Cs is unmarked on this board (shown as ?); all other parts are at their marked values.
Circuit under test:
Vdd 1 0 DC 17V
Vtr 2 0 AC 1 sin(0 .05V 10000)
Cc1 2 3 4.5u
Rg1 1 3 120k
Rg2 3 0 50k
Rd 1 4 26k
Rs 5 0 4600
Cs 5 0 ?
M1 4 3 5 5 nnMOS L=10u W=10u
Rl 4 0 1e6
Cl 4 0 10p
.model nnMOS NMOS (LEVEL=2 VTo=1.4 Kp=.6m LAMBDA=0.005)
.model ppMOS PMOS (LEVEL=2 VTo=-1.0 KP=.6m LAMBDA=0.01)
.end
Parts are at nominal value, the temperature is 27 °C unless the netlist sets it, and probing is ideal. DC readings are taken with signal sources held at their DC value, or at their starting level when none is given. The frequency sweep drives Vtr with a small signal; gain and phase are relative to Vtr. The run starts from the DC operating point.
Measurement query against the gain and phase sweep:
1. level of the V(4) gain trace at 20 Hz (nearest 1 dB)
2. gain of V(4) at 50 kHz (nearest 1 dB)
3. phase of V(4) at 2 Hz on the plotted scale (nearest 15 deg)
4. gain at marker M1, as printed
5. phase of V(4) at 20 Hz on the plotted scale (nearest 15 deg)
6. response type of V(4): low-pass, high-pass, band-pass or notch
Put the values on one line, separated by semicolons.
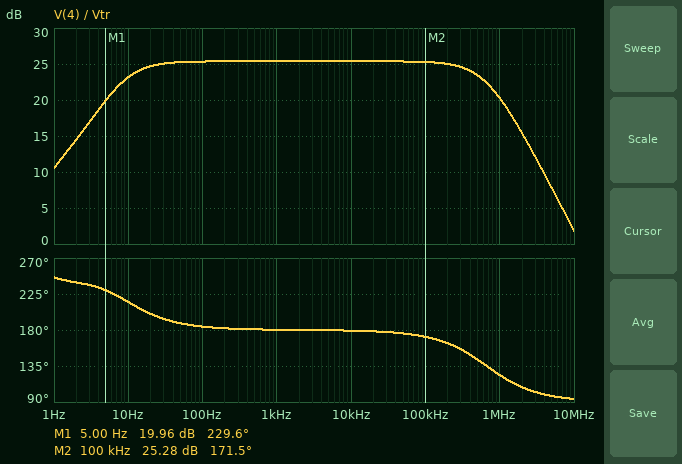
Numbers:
25 dB; 25 dB; 240 deg; 19.96 dB; 195 deg; band-pass
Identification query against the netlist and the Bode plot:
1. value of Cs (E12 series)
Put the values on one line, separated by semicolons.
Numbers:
18 µF
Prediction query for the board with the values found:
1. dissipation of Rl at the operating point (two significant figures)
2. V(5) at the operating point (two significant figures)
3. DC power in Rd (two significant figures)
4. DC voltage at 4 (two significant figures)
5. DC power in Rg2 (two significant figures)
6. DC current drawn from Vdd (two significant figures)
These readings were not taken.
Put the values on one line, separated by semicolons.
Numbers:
15 µW; 2.3 V; 6.7 mW; 3.8 V; 500 µW; 610 µA
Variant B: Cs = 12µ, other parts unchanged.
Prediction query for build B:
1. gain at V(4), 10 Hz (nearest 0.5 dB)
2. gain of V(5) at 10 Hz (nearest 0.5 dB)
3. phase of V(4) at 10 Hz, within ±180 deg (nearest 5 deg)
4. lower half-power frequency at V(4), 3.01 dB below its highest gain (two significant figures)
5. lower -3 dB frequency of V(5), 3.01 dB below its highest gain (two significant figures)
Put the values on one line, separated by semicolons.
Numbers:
21.5 dB; -4.5 dB; -140 deg; 12 Hz; 870 mHz
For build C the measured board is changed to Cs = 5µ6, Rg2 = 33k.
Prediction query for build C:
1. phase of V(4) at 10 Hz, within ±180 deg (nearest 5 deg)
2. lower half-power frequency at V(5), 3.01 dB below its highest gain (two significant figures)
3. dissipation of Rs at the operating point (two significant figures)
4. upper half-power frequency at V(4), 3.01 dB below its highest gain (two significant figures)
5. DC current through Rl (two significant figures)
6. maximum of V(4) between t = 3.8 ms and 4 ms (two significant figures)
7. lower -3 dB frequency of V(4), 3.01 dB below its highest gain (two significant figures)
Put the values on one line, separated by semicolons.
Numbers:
-140 deg; 1.2 Hz; 370 µW; 650 kHz; 9.3 µA; 10 V; 21 Hz
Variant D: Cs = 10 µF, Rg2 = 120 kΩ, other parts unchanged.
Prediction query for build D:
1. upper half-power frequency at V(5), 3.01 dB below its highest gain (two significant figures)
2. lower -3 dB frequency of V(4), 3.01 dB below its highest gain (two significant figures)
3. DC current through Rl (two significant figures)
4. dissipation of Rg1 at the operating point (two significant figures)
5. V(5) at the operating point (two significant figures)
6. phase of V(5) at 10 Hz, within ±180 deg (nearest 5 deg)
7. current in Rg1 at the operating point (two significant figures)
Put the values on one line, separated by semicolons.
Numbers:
5.2 Hz; 880 mHz; 2.7 µA; 600 µW; 2.5 V; -65 deg; 71 µA
